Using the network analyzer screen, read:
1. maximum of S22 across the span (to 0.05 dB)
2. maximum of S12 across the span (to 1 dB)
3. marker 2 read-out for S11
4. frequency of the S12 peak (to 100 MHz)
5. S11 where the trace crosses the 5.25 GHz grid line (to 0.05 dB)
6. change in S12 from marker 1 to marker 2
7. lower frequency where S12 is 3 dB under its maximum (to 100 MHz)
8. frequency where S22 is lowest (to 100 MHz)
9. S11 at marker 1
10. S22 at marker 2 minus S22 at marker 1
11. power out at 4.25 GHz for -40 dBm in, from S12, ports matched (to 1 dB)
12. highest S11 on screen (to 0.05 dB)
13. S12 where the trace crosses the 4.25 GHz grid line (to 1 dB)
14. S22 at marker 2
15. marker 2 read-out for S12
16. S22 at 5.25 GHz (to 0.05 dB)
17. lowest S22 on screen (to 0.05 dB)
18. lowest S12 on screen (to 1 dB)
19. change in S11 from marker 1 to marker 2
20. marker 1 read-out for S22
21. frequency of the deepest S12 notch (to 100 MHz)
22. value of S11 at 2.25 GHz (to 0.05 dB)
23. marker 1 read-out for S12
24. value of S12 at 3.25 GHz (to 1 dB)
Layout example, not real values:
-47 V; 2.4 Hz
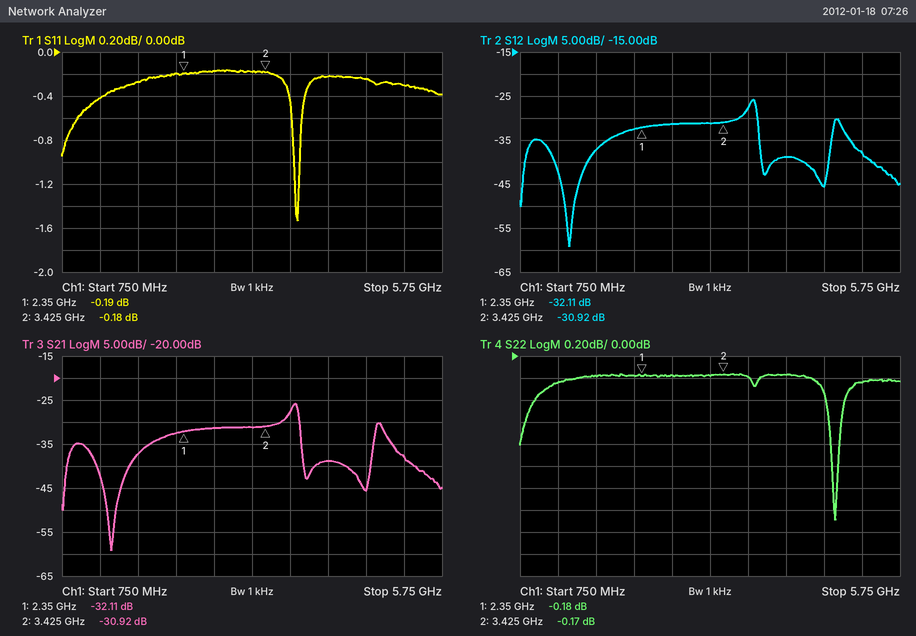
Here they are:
-0.15 dB; -26 dB; -0.18 dB; 3.8 GHz; -0.30 dB; 1.19 dB; 3.7 GHz; 4.9 GHz; -0.19 dB; 0.01 dB; -79 dBm; -0.15 dB; -39 dB; -0.17 dB; -30.92 dB; -0.25 dB; -1.50 dB; -59 dB; 0.01 dB; -0.18 dB; 1.4 GHz; -0.20 dB; -32.11 dB; -31 dB
